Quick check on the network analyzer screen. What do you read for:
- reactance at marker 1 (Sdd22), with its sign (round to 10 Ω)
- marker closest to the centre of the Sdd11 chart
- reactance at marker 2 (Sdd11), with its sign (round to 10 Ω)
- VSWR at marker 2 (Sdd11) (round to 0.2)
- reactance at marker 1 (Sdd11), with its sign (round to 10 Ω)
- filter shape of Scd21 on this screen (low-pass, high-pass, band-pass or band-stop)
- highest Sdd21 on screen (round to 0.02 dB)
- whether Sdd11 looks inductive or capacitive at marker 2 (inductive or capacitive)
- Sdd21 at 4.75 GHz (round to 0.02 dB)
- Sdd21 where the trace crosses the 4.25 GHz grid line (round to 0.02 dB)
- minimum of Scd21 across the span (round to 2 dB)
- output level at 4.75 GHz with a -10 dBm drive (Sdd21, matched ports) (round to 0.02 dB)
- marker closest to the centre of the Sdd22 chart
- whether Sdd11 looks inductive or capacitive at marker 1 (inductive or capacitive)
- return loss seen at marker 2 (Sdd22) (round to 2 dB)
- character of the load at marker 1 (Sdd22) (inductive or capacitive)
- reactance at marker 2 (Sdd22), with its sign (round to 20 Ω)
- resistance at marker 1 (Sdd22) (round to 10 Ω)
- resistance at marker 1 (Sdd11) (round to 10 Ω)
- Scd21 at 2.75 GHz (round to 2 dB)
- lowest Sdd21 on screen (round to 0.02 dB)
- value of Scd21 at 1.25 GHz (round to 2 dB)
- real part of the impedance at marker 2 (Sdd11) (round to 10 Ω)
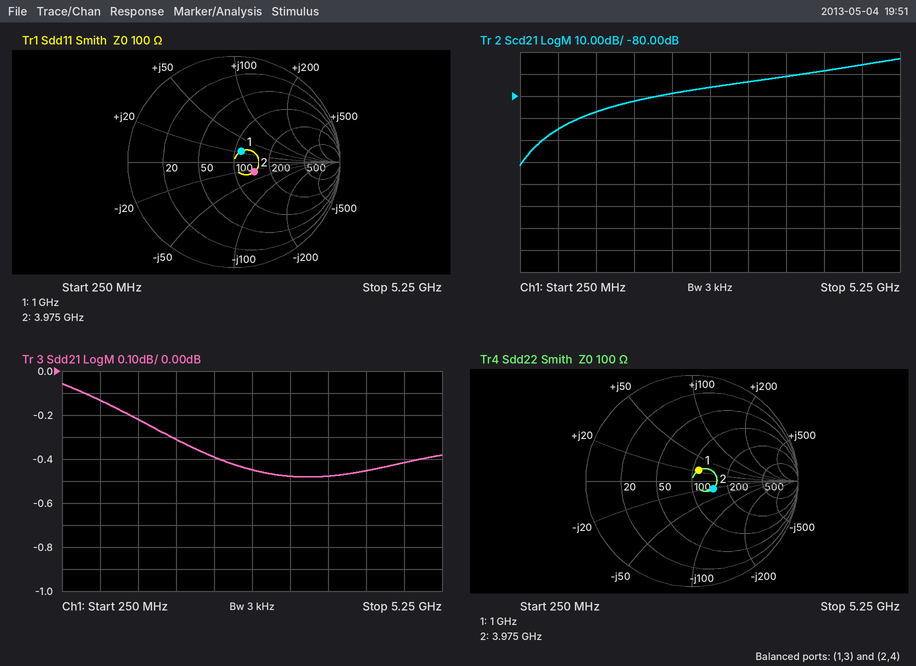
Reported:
+20 Ω
marker 1
-30 Ω
1.6
+20 Ω
high-pass
-0.06 dB
capacitive
-0.42 dB
-0.46 dB
-112 dB
-10.42 dBm
marker 1
inductive
14 dB
inductive
-20 Ω
110 Ω
110 Ω
-76 dB
-0.48 dB
-88 dB
140 Ω
